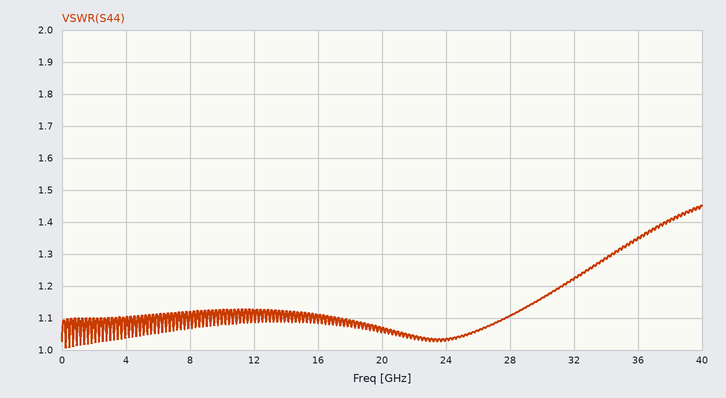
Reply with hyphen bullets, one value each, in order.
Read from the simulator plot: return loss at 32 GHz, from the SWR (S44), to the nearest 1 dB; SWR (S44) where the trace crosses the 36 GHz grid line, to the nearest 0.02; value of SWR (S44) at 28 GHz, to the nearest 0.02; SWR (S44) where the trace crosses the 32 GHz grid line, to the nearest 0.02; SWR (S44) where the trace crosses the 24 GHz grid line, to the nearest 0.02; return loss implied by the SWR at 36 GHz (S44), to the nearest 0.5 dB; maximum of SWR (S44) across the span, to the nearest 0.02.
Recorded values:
- 20 dB
- 1.36
- 1.10
- 1.22
- 1.04
- 16.5 dB
- 1.46
